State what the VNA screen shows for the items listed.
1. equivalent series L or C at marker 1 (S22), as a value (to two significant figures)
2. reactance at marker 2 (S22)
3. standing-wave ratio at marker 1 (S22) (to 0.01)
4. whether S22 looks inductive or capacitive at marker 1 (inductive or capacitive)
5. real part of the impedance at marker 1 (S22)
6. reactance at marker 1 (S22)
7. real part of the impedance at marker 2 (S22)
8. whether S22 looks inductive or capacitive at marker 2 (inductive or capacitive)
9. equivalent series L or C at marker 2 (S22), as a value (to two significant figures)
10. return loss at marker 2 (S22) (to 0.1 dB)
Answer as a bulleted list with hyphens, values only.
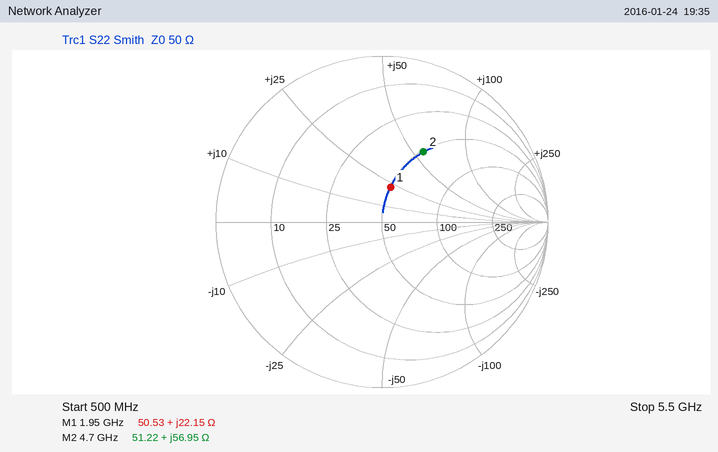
- 1.8 nH
- +56.95 Ω
- 1.55
- inductive
- 50.53 Ω
- +22.15 Ω
- 51.22 Ω
- inductive
- 1.9 nH
- 6.2 dB
